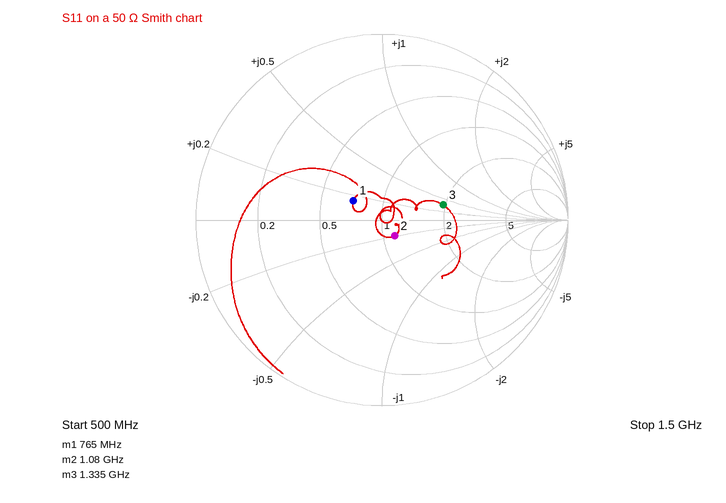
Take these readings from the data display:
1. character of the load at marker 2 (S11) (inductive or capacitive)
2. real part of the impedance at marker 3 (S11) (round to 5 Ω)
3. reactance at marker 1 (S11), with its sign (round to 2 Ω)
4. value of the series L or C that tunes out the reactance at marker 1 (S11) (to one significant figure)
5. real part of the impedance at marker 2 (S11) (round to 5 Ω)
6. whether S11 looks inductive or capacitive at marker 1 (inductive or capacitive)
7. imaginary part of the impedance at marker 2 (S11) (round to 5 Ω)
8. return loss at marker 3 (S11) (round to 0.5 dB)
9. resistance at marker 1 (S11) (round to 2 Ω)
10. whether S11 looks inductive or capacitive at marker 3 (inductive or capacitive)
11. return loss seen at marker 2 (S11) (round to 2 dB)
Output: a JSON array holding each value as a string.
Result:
["capacitive", "95 Ω", "+8 Ω", "30 pF", "55 Ω", "inductive", "-10 Ω", "9.5 dB", "36 Ω", "inductive", "20 dB"]
